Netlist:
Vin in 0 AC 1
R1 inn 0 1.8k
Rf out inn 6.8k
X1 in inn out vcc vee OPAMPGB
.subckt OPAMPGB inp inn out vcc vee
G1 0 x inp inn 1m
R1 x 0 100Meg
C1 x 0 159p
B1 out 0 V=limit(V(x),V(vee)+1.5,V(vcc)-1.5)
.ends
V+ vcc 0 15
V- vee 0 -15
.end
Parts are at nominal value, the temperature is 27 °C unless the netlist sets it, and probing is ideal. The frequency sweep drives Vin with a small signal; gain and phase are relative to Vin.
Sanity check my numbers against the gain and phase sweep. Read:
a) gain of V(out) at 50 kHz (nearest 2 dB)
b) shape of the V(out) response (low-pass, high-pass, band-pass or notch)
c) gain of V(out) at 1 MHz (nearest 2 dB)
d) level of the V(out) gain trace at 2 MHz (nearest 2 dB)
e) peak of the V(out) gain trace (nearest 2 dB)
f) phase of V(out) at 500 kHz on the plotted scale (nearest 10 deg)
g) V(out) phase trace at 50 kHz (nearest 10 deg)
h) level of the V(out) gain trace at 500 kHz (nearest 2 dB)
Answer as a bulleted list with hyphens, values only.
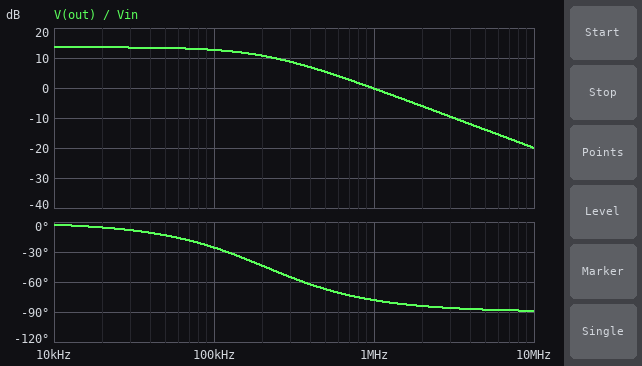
- 14 dB
- low-pass
- 0 dB
- -6 dB
- 14 dB
- -70 deg
- -10 deg
- 6 dB
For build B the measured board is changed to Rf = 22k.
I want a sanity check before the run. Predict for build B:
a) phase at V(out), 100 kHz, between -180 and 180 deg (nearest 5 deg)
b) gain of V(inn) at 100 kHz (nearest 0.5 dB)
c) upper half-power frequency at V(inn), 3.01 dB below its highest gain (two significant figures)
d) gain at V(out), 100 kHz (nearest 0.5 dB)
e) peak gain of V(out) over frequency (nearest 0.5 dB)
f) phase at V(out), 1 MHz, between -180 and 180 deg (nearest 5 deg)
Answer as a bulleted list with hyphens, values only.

- -55 deg
- -4.5 dB
- 76 kHz
- 18.0 dB
- 22.5 dB
- -85 deg
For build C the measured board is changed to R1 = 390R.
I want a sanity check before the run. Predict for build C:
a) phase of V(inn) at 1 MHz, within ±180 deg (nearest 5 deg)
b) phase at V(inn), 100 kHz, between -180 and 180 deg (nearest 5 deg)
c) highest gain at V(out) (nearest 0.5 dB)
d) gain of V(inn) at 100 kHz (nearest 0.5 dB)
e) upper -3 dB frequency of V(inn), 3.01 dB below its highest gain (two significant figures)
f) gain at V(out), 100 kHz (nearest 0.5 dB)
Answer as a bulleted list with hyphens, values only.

- -85 deg
- -60 deg
- 25.5 dB
- -6.5 dB
- 54 kHz
- 19.0 dB
